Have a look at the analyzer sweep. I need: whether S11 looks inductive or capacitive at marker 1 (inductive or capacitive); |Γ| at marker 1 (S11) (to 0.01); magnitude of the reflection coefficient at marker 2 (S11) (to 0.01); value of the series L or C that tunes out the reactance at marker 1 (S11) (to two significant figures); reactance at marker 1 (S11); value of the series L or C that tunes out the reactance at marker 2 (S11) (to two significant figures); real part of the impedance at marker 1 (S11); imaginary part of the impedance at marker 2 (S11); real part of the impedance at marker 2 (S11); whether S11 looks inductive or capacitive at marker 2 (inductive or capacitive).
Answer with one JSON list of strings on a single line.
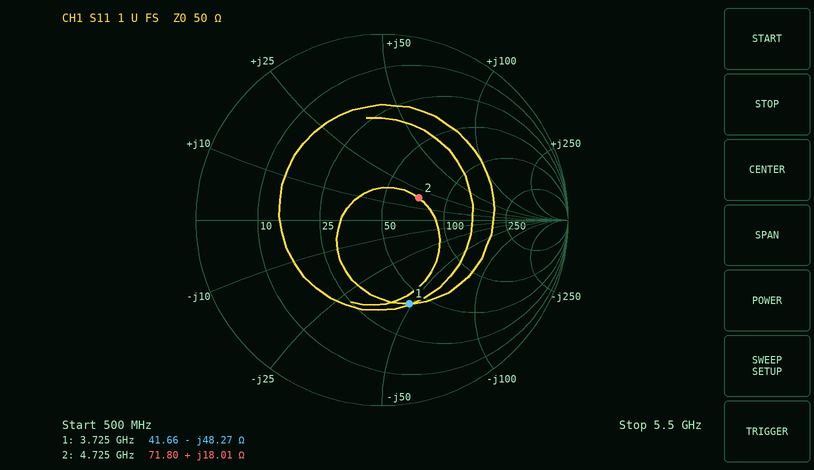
["capacitive", "0.47", "0.23", "2.1 nH", "-48.27 Ω", "1.9 pF", "41.66 Ω", "+18.01 Ω", "71.80 Ω", "inductive"]
